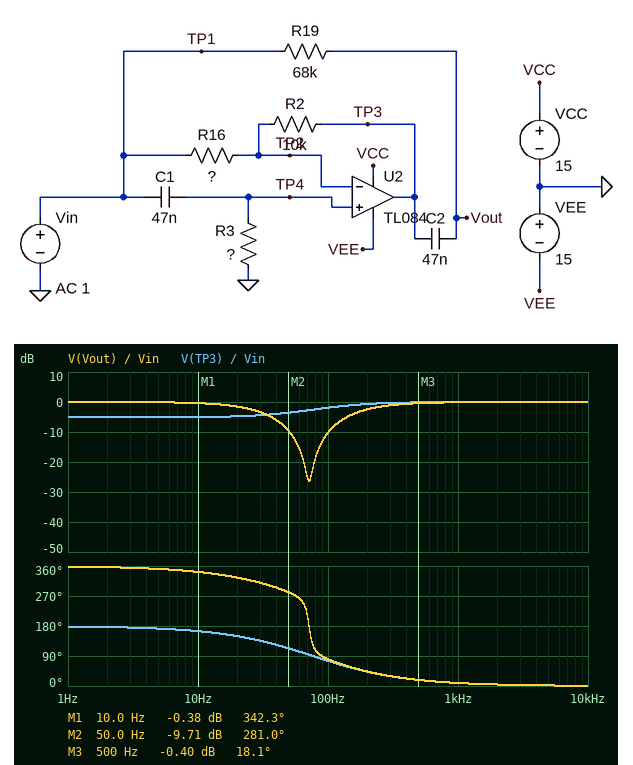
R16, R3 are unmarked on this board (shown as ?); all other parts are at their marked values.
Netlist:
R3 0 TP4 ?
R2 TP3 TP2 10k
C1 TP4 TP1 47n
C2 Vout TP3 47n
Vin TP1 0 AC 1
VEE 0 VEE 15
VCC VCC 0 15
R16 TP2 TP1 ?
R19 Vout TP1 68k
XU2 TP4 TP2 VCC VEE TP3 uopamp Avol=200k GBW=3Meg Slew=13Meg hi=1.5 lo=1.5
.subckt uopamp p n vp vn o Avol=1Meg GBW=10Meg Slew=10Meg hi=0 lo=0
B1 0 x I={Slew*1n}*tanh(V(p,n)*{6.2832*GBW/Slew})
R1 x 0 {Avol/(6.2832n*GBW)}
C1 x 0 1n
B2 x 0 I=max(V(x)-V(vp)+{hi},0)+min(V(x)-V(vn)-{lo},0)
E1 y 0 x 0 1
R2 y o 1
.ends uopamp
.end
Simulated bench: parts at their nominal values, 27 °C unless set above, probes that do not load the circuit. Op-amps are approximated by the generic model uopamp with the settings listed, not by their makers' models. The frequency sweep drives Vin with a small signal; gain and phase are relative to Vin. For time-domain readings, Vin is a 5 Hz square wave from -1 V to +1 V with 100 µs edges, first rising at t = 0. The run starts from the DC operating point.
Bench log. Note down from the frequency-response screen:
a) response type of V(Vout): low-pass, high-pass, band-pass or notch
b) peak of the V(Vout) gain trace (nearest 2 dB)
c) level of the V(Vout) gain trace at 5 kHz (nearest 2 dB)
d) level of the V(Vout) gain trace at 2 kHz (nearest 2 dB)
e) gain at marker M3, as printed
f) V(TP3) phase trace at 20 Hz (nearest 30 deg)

notch
0 dB
0 dB
0 dB
-0.40 dB
150 deg
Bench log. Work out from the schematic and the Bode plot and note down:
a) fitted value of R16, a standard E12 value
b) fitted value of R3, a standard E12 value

18 kΩ
33 kΩ
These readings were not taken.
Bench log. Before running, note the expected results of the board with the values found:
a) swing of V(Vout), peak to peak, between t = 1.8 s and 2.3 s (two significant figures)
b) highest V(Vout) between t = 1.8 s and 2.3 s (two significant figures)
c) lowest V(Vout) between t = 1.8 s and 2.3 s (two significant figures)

2.0 V
1.0 V
-1.0 V
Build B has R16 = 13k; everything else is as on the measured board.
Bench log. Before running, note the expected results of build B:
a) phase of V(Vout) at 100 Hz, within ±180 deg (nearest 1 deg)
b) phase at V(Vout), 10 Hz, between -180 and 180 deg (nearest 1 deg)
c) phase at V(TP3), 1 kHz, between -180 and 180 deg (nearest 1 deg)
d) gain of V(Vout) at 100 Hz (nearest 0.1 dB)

103 deg
-20 deg
10 deg
-9.0 dB
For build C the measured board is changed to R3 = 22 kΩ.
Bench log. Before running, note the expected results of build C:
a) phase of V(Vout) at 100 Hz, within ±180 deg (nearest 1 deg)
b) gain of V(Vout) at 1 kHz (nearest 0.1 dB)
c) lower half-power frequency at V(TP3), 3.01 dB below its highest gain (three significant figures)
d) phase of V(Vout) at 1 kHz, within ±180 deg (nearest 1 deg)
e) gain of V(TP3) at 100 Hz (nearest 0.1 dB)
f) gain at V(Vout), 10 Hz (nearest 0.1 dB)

140 deg
-0.2 dB
95.2 Hz
14 deg
-2.9 dB
-0.3 dB
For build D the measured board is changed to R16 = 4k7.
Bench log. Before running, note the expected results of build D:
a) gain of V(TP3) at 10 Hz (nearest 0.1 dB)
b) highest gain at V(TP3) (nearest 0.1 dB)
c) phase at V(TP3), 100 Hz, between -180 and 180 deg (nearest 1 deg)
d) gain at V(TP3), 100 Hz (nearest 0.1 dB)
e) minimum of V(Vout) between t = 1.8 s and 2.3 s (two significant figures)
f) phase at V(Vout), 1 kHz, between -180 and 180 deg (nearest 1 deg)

6.5 dB
6.6 dB
111 deg
4.5 dB
-2.2 V
18 deg
